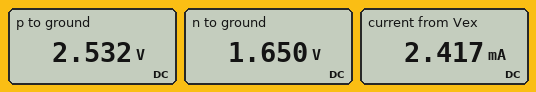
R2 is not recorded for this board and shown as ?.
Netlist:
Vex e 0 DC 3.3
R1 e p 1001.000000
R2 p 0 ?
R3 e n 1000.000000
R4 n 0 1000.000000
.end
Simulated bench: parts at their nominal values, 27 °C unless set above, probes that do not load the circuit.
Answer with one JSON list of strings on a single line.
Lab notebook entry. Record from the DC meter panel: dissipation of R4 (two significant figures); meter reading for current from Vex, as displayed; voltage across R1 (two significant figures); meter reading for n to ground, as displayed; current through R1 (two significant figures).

["2.7 mW", "2.417 mA", "770 mV", "1.650 V", "770 µA"]
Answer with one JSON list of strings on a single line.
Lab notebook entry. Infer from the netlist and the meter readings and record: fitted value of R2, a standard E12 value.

["3.3 kΩ"]
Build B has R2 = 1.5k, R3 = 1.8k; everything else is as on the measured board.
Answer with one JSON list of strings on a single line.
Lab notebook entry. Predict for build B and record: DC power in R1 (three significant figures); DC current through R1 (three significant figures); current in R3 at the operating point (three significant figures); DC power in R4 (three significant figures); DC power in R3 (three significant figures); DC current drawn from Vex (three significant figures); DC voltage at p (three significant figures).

["1.74 mW", "1.32 mA", "1.18 mA", "1.39 mW", "2.50 mW", "2.50 mA", "1.98 V"]
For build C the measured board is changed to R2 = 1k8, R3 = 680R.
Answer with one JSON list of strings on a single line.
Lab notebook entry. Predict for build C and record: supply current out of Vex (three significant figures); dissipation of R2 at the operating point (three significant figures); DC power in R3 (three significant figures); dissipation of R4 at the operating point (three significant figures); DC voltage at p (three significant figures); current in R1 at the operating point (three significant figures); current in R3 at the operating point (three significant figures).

["3.14 mA", "2.50 mW", "2.62 mW", "3.86 mW", "2.12 V", "1.18 mA", "1.96 mA"]
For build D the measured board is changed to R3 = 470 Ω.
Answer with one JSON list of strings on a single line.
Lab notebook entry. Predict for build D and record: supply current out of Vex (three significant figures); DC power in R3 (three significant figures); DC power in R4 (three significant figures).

["3.01 mA", "2.37 mW", "5.04 mW"]
